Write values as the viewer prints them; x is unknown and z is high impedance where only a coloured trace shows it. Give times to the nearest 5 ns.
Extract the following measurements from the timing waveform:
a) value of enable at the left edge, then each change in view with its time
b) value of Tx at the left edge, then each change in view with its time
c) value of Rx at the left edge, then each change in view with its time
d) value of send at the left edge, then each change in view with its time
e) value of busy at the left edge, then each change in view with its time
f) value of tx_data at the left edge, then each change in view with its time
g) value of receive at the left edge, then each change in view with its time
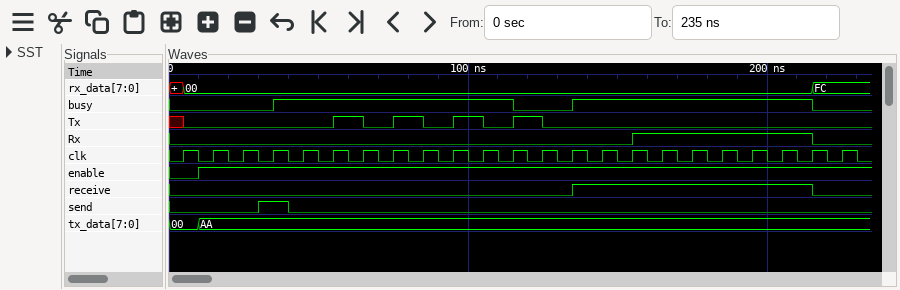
0, 1 at 10 ns
x, 0 at 5 ns, 1 at 55 ns, 0 at 65 ns, 1 at 75 ns, 0 at 85 ns, 1 at 95 ns, 0 at 105 ns, 1 at 115 ns, 0 at 125 ns
0, 1 at 155 ns, 0 at 215 ns
0, 1 at 30 ns, 0 at 40 ns
0, 1 at 35 ns, 0 at 115 ns, 1 at 135 ns, 0 at 215 ns
00, AA at 10 ns
0, 1 at 135 ns, 0 at 215 ns
